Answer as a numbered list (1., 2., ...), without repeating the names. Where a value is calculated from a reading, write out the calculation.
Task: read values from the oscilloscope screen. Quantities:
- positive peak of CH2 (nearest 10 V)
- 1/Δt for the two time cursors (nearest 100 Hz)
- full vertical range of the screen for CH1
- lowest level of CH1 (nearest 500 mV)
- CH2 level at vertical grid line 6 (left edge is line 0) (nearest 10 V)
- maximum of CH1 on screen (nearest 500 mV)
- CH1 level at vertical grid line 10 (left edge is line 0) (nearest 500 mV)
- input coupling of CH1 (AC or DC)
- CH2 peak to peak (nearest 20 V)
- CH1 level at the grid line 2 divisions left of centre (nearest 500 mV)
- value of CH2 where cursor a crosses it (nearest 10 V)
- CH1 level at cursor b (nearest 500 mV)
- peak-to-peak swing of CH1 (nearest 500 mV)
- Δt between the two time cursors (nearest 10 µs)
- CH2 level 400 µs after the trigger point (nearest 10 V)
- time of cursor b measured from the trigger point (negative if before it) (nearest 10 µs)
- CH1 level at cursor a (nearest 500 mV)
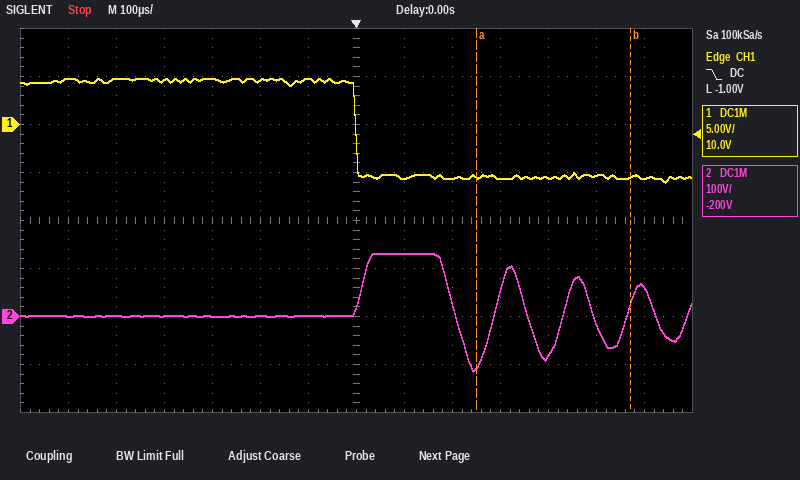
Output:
1. 130 V
2. 1 / 320 µs ≈ 3.1 kHz
3. 40 V
4. -6.0 V
5. 0 V
6. 5.0 V
7. -5.5 V
8. DC
9. 240 V
10. 4.5 V
11. -100 V
12. -5.5 V
13. 5.0 V − (-6.0 V) = 11.0 V
14. 320 µs
15. -80 V
16. +570 µs
17. -5.5 V
